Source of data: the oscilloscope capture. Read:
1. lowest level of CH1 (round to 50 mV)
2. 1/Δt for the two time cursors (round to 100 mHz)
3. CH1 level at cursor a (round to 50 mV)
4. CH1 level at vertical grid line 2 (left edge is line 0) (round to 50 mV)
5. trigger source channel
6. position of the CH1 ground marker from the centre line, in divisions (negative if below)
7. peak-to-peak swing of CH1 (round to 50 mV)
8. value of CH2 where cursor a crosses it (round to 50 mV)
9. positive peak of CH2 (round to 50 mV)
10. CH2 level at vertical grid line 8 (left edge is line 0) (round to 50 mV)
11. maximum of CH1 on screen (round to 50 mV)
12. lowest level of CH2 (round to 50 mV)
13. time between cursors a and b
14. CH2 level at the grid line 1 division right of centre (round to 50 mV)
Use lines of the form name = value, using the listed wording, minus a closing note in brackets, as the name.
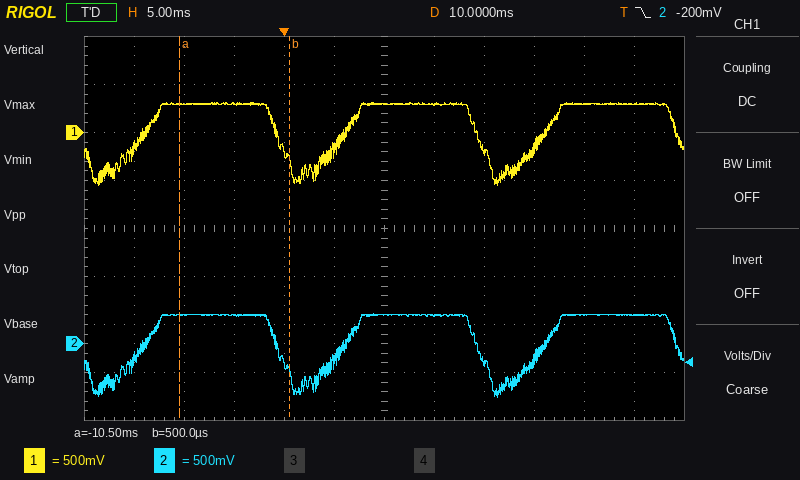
lowest level of CH1 = -550 mV
1/Δt for the two time cursors = 90.9 Hz
CH1 level at cursor a = 300 mV
CH1 level at vertical grid line 2 (left edge is line 0) = 300 mV
trigger source channel = CH2
position of the CH1 ground marker from the centre line, in divisions = +2.0 div
peak-to-peak swing of CH1 = 850 mV
value of CH2 where cursor a crosses it = 300 mV
positive peak of CH2 = 300 mV
CH2 level at vertical grid line 8 (left edge is line 0) = -200 mV
maximum of CH1 on screen = 300 mV
lowest level of CH2 = -550 mV
time between cursors a and b = 11.0 ms
CH2 level at the grid line 1 division right of centre = 300 mV
